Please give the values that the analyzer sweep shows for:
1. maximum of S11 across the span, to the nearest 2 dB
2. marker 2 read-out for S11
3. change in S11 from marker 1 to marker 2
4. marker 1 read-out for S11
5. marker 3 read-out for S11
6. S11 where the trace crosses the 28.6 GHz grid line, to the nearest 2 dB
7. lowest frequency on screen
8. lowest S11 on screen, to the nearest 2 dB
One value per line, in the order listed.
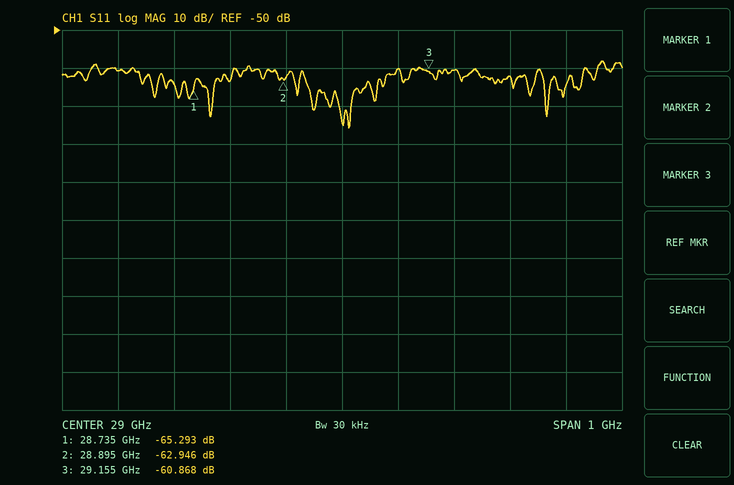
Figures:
-58 dB
-62.946 dB
2.347 dB
-65.293 dB
-60.868 dB
-60 dB
28.5 GHz
-76 dB
